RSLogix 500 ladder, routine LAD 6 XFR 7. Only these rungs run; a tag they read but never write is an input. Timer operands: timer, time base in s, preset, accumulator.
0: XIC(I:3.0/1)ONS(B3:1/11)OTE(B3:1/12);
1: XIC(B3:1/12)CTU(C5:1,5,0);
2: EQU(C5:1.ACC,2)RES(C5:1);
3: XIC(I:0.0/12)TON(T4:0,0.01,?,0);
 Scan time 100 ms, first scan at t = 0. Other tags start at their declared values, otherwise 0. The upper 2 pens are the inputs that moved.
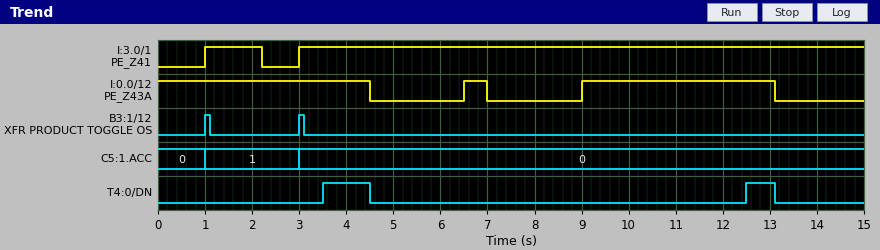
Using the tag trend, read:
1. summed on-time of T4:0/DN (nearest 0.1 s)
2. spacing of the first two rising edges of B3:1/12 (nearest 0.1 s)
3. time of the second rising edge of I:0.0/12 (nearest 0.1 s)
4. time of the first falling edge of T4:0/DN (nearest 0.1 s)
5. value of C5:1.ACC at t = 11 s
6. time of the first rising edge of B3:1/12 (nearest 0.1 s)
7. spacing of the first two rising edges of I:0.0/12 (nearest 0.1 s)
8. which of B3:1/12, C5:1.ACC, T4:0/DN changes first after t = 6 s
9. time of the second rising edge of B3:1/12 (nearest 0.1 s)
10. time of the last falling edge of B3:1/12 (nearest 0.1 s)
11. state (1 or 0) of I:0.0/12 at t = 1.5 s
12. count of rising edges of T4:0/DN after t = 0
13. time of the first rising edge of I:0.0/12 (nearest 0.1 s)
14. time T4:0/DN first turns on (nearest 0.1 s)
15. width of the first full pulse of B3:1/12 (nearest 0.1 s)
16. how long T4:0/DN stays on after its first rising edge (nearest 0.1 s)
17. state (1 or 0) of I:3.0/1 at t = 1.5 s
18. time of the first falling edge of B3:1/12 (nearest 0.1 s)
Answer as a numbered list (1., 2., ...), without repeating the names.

1. 1.6 s
2. 2.0 s
3. 9.0 s
4. 4.5 s
5. 0
6. 1.0 s
7. 2.5 s
8. T4:0/DN
9. 3.0 s
10. 3.1 s
11. 1
12. 2
13. 6.5 s
14. 3.5 s
15. 0.1 s
16. 1.0 s
17. 1
18. 1.1 s
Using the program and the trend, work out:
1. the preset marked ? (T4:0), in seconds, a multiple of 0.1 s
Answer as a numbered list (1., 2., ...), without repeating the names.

1. 3.5 s
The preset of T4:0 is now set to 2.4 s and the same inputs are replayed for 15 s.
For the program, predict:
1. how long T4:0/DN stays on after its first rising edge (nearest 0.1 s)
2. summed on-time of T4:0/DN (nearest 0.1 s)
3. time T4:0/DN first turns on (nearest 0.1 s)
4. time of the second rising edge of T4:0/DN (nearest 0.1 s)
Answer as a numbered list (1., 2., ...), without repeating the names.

1. 2.1 s
2. 3.8 s
3. 2.4 s
4. 11.4 s
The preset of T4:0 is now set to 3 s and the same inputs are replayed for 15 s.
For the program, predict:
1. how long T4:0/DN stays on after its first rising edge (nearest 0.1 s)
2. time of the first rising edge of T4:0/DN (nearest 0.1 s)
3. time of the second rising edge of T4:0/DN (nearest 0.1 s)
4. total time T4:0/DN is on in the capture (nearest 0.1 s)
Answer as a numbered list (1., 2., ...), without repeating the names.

1. 1.5 s
2. 3.0 s
3. 12.0 s
4. 2.6 s
